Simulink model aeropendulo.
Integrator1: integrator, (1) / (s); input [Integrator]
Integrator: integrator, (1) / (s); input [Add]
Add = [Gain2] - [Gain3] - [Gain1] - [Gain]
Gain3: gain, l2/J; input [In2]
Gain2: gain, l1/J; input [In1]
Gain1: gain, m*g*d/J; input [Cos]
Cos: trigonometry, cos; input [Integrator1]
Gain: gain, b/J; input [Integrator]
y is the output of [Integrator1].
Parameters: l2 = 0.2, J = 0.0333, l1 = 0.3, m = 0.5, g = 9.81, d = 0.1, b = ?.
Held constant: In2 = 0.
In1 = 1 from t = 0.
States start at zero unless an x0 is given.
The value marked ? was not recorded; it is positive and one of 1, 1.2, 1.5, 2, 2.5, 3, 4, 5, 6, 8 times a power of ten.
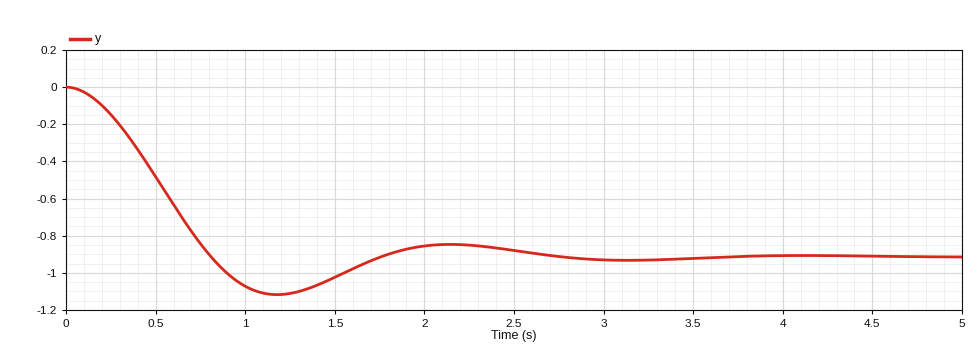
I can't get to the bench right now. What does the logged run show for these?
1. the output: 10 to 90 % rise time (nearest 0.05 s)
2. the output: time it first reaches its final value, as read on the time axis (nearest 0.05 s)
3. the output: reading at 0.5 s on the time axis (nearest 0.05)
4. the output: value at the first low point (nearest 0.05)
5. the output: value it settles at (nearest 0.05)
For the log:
0.55 s
0.80 s
-0.50
-1.10
-0.90
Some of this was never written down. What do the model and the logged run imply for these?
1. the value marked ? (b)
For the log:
0.08
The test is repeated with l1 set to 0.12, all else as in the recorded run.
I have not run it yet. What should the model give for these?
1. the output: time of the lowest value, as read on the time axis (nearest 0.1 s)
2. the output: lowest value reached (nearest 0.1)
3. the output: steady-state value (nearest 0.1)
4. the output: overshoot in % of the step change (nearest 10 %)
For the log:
1.0 s
-1.7
-1.3
30 %
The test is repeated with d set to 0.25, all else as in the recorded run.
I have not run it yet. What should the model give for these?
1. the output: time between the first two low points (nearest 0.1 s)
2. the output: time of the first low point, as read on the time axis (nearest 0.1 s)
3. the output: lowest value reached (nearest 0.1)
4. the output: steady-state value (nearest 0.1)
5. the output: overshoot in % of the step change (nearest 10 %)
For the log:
1.1 s
0.6 s
-1.9
-1.3
40 %
